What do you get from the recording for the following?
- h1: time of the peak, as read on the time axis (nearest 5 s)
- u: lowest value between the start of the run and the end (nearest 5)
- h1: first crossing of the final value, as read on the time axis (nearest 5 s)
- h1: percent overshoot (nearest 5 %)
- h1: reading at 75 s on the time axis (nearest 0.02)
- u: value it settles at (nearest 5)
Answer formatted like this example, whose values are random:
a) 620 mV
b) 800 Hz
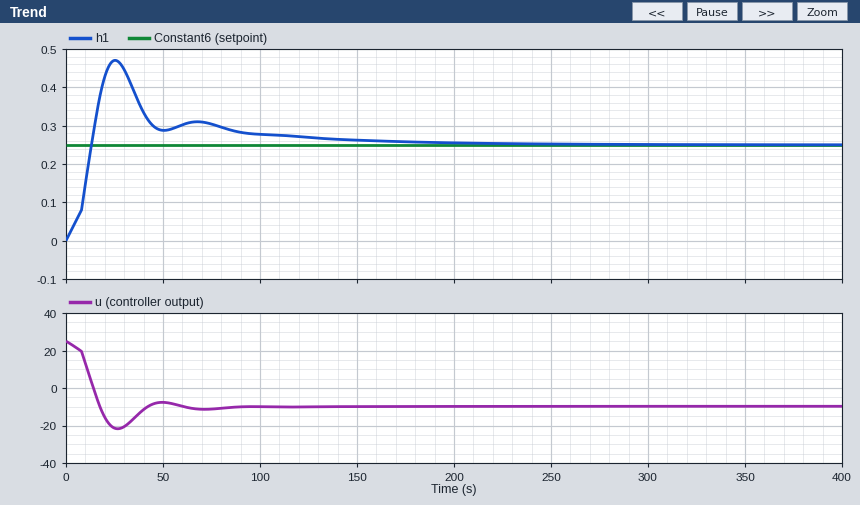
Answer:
a) 25 s
b) -20
c) 15 s
d) 90 %
e) 0.30
f) -10
